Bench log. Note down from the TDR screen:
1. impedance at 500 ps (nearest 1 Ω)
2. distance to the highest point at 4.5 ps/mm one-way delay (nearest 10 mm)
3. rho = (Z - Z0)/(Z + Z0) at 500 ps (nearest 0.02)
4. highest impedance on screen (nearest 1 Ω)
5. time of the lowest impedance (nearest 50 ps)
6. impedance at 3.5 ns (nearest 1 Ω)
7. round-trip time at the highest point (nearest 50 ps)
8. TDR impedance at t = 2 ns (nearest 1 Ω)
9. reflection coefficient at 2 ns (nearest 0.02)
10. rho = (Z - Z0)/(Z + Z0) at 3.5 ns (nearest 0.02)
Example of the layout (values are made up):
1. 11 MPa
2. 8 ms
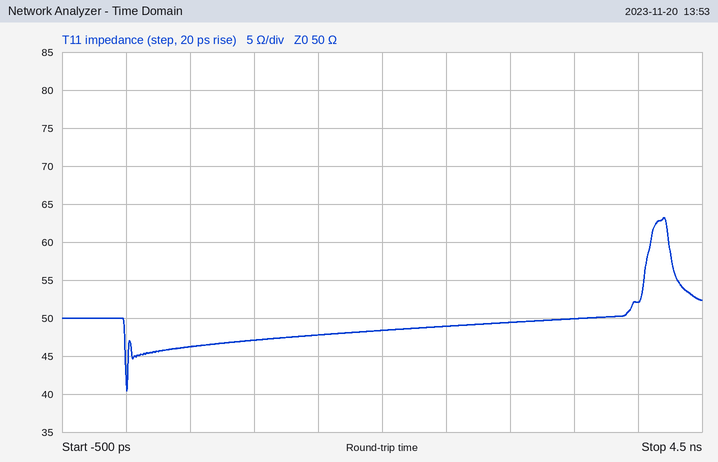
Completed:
1. 46 Ω
2. 470 mm
3. -0.04
4. 63 Ω
5. 0 ps
6. 50 Ω
7. 4.20 ns
8. 48 Ω
9. -0.02
10. 0.00
